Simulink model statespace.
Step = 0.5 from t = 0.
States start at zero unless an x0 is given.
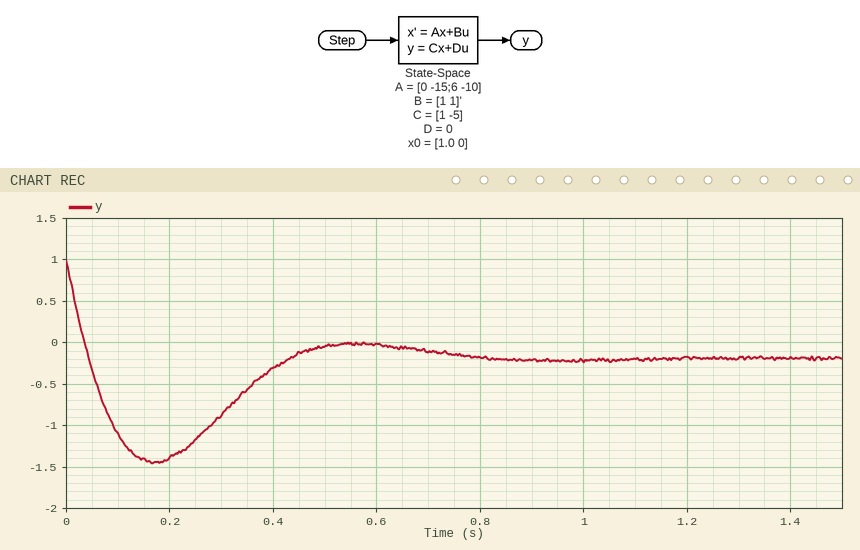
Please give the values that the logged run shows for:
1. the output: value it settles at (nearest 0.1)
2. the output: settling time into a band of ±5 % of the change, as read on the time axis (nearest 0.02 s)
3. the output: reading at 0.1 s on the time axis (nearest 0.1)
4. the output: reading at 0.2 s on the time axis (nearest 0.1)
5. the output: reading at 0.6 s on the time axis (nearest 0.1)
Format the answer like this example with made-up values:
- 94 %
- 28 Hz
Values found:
- -0.2
- 0.74 s
- -1.1
- -1.4
- 0.0
